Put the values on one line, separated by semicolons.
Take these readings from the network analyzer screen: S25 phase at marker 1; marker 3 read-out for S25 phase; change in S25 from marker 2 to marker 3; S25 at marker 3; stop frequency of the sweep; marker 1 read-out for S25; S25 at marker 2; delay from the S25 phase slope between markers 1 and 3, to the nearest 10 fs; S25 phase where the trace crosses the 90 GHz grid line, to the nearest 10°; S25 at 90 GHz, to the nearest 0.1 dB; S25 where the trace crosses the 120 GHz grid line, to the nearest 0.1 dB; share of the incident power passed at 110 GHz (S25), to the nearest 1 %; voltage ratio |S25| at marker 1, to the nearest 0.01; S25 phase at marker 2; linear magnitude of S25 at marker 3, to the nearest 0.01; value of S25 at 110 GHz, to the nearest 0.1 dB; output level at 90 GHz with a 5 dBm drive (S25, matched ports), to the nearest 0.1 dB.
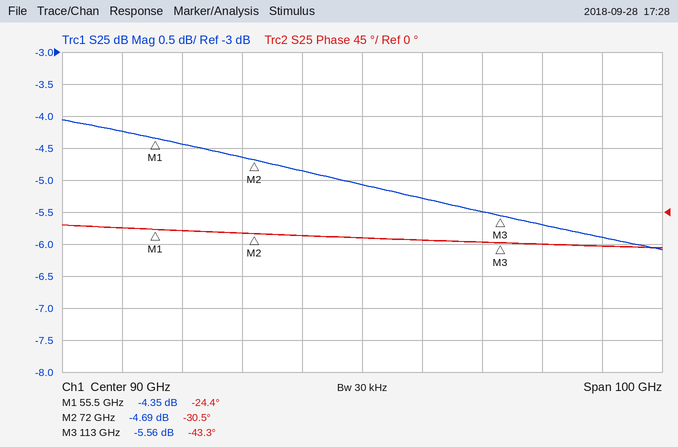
-24.4°; -43.3°; -0.87 dB; -5.56 dB; 140 GHz; -4.35 dB; -4.69 dB; 910 fs; -40°; -5.1 dB; -5.7 dB; 28 %; 0.61; -30.5°; 0.53; -5.5 dB; -0.1 dBm
